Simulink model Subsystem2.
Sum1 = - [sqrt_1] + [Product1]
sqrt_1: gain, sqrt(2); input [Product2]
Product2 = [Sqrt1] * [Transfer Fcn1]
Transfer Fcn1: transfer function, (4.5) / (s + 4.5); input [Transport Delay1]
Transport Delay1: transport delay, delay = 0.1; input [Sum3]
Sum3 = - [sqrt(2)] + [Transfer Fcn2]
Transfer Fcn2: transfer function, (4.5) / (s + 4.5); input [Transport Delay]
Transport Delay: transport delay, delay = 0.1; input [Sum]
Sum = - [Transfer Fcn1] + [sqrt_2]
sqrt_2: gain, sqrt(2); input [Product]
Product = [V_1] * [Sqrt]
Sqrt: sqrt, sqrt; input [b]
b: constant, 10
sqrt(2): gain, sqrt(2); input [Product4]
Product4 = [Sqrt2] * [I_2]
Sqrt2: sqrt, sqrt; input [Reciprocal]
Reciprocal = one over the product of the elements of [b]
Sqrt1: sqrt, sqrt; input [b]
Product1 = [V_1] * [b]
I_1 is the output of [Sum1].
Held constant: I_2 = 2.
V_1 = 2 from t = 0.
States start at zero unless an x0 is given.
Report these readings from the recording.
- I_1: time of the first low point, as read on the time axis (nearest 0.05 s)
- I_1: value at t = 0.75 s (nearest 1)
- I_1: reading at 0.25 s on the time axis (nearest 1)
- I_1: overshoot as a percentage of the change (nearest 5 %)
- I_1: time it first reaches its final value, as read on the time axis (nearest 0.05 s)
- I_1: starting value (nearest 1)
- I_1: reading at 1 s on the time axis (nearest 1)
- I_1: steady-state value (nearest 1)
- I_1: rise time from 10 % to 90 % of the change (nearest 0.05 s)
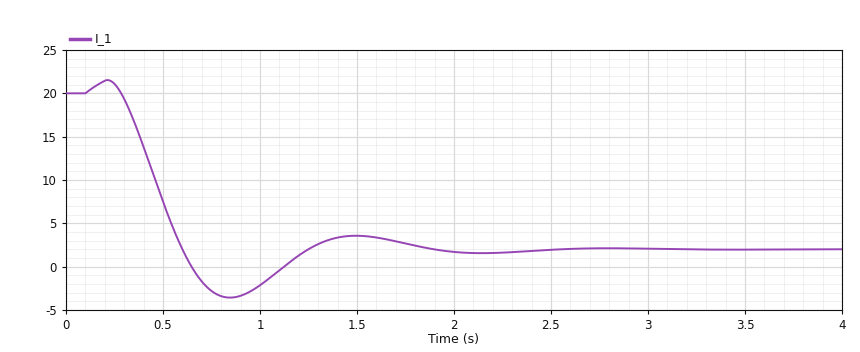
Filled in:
0.85 s
-3
21
30 %
0.60 s
20
-2
2
0.25 s
